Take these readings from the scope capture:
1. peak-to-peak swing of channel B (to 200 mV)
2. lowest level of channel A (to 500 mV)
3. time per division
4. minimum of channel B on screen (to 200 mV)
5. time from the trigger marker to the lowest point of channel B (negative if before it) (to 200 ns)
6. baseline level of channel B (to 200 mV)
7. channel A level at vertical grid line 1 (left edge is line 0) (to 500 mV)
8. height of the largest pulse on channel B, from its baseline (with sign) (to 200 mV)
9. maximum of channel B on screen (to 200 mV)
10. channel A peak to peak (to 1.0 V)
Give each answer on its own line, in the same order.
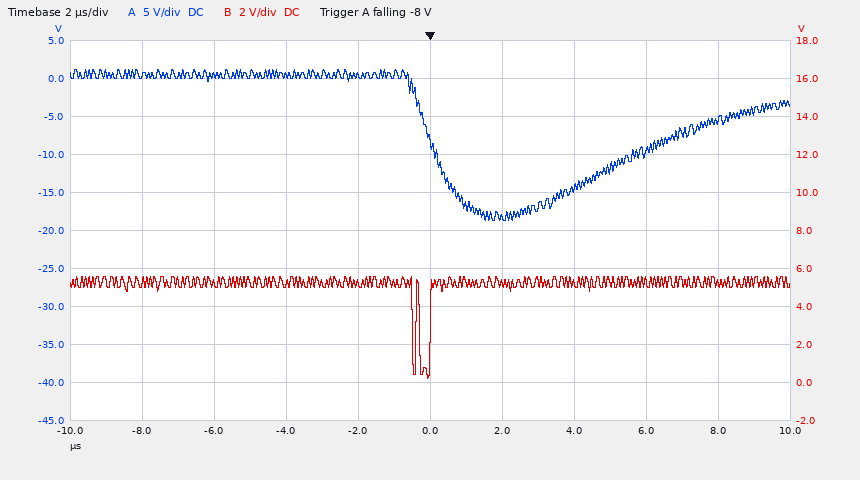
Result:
5.4 V
-18.5 V
2 µs
200 mV
0.0 µs
5.2 V
500 mV
-5.0 V
5.6 V
20.0 V
